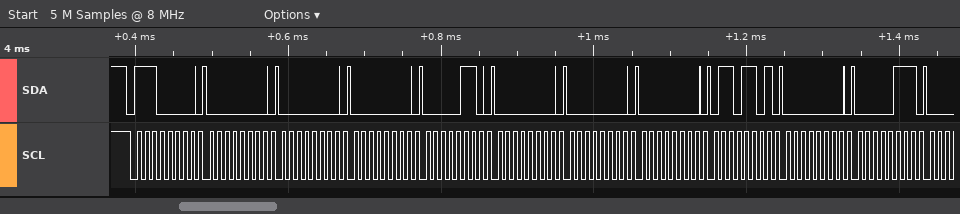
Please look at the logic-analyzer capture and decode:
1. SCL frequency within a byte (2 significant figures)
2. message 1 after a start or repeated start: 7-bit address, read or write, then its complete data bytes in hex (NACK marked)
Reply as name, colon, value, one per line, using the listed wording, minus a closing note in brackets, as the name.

SCL frequency within a byte: 100 kHz
message 1 after a start or repeated start: 7-bit address, read or write, then its complete data bytes in hex: 0x70 write: 00 00 00 06 00 00 00 6D 00 07
